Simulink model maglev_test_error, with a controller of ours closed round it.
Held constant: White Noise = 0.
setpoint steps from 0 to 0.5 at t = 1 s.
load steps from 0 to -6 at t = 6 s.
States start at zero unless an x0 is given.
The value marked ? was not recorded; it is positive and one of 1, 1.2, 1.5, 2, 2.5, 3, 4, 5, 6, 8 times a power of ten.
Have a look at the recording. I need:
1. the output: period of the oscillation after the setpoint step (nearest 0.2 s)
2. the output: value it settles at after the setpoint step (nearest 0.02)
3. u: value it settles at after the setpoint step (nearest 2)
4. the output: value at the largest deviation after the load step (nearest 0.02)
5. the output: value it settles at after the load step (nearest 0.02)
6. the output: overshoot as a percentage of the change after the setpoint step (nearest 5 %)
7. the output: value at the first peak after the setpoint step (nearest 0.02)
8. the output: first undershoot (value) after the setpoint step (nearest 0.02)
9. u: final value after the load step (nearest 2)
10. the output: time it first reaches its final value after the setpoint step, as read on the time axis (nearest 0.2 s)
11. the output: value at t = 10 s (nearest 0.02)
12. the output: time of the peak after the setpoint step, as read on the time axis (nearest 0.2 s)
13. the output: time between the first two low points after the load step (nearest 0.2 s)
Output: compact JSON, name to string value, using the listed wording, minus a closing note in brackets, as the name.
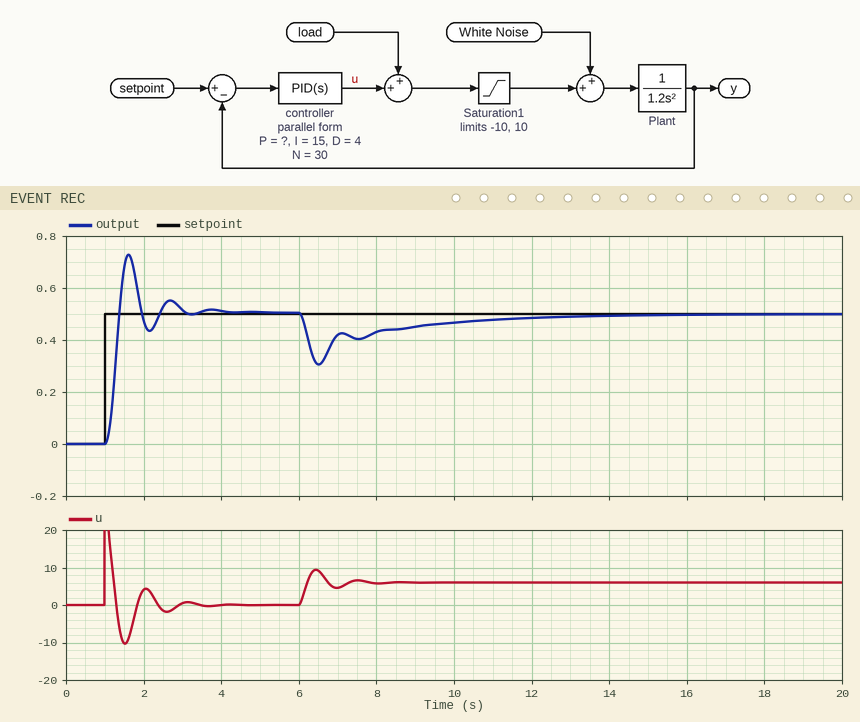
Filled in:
{"the output: period of the oscillation after the setpoint step": "1.0 s", "the output: value it settles at after the setpoint step": "0.50", "u: value it settles at after the setpoint step": "0", "the output: value at the largest deviation after the load step": "0.30", "the output: value it settles at after the load step": "0.50", "the output: overshoot as a percentage of the change after the setpoint step": "45 %", "the output: value at the first peak after the setpoint step": "0.72", "the output: first undershoot (value) after the setpoint step": "0.44", "u: final value after the load step": "6", "the output: time it first reaches its final value after the setpoint step, as read on the time axis": "1.4 s", "the output: value at t = 10 s": "0.46", "the output: time of the peak after the setpoint step, as read on the time axis": "1.6 s", "the output: time between the first two low points after the load step": "1.0 s"}
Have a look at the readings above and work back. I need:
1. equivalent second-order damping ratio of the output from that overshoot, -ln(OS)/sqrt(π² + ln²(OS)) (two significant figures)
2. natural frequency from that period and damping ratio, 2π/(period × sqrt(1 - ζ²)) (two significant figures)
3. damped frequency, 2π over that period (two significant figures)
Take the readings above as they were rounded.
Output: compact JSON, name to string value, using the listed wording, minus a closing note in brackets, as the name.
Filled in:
{"equivalent second-order damping ratio of the output from that overshoot, -ln(OS)/sqrt(π² + ln²(OS))": "0.25", "natural frequency from that period and damping ratio, 2π/(period × sqrt(1 - ζ²))": "6.5 rad/s", "damped frequency, 2π over that period": "6.3 rad/s"}
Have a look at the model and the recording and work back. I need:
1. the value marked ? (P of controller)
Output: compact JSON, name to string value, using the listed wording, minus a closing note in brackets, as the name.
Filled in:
{"the value marked ?": "40"}
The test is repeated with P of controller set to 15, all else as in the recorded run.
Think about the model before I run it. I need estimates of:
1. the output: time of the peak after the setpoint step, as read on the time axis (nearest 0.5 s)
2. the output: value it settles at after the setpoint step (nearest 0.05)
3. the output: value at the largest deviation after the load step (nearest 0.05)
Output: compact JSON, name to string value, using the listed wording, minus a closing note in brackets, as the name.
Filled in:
{"the output: time of the peak after the setpoint step, as read on the time axis": "2.0 s", "the output: value it settles at after the setpoint step": "0.50", "the output: value at the largest deviation after the load step": "0.10"}
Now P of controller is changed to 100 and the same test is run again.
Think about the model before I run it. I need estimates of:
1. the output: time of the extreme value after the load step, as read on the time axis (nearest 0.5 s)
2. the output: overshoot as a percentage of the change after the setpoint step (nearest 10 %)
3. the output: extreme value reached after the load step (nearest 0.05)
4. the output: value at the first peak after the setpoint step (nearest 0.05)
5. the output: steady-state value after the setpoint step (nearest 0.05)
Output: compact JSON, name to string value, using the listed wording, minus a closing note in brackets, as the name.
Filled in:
{"the output: time of the extreme value after the load step, as read on the time axis": "6.5 s", "the output: overshoot as a percentage of the change after the setpoint step": "70 %", "the output: extreme value reached after the load step": "0.40", "the output: value at the first peak after the setpoint step": "0.85", "the output: steady-state value after the setpoint step": "0.50"}
